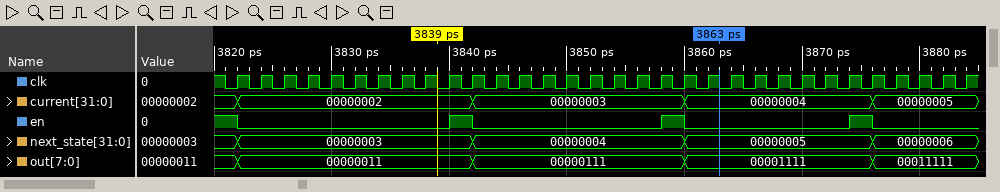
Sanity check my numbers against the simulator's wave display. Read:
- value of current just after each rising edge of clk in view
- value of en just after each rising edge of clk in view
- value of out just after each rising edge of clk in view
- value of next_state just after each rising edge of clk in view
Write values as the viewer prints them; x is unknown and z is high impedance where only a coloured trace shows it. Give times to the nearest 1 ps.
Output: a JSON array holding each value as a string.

["00000002, 00000002, 00000002, 00000002, 00000002, 00000002, 00000002, 00000002, 00000002, 00000002, 00000003, 00000003, 00000003, 00000003, 00000003, 00000003, 00000003, 00000003, 00000003, 00000004, 00000004, 00000004, 00000004, 00000004, 00000004, 00000004, 00000004, 00000005, 00000005, 00000005, 00000005, 00000005", "0 0 0 0 0 0 0 0 0 1 0 0 0 0 0 0 0 0 1 0 0 0 0 0 0 0 1 0 0 0 0 0", "00000011, 00000011, 00000011, 00000011, 00000011, 00000011, 00000011, 00000011, 00000011, 00000011, 00000111, 00000111, 00000111, 00000111, 00000111, 00000111, 00000111, 00000111, 00000111, 00001111, 00001111, 00001111, 00001111, 00001111, 00001111, 00001111, 00001111, 00011111, 00011111, 00011111, 00011111, 00011111", "00000003, 00000003, 00000003, 00000003, 00000003, 00000003, 00000003, 00000003, 00000003, 00000003, 00000004, 00000004, 00000004, 00000004, 00000004, 00000004, 00000004, 00000004, 00000004, 00000005, 00000005, 00000005, 00000005, 00000005, 00000005, 00000005, 00000005, 00000006, 00000006, 00000006, 00000006, 00000006"]
